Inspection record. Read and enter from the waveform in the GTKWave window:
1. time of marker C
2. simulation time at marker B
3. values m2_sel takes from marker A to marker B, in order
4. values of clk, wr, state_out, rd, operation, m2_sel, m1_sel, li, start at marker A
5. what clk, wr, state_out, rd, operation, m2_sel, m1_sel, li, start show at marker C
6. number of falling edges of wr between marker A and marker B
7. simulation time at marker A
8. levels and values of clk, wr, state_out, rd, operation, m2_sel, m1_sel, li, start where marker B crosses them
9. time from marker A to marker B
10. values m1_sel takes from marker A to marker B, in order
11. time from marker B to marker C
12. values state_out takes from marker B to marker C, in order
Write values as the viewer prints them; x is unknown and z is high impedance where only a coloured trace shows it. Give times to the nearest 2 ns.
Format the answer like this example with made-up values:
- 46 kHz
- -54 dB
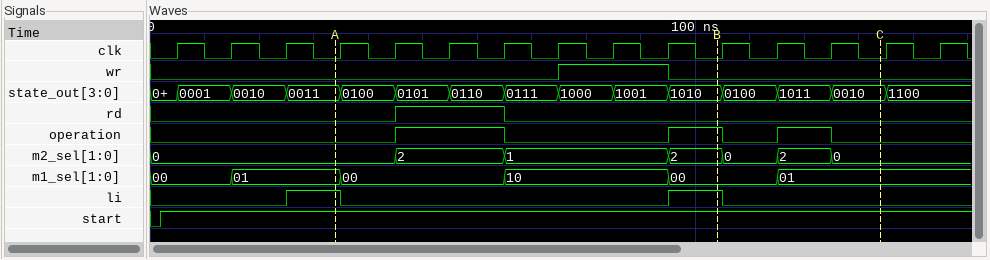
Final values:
- 134 ns
- 104 ns
- 0, 2, 1, 2
- clk=0, wr=0, state_out=0011, rd=0, operation=0, m2_sel=0, m1_sel=01, li=1, start=1
- clk=0, wr=0, state_out=0010, rd=0, operation=0, m2_sel=0, m1_sel=01, li=0, start=1
- 1
- 34 ns
- clk=0, wr=0, state_out=1010, rd=0, operation=1, m2_sel=2, m1_sel=00, li=1, start=1
- 70 ns
- 01, 00, 10, 00
- 30 ns
- 1010, 0100, 1011, 0010
